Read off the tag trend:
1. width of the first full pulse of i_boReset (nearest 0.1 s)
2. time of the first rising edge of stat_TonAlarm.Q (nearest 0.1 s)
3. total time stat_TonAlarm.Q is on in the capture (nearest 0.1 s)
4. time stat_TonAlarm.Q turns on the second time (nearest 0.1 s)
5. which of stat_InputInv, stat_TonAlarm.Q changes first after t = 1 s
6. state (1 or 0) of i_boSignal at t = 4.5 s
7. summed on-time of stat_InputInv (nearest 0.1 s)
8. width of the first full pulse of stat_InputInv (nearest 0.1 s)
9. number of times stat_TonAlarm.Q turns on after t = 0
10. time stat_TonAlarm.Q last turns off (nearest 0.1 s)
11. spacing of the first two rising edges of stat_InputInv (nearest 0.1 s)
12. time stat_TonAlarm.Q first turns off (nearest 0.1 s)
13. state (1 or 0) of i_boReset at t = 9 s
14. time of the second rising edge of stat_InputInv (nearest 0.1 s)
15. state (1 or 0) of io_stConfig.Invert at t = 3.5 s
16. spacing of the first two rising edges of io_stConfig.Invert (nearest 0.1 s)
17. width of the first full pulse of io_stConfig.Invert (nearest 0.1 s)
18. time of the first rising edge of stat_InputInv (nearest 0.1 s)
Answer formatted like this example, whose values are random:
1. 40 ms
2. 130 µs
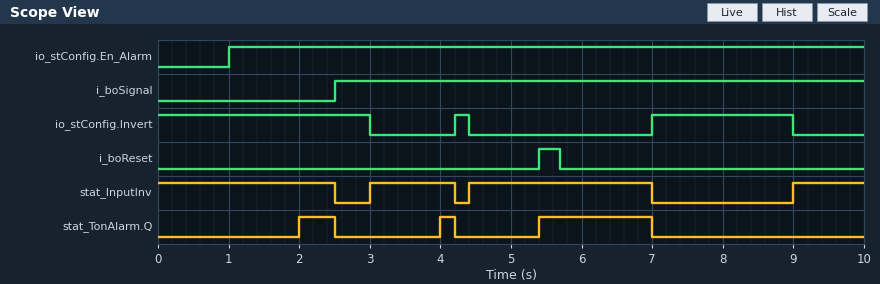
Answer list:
1. 0.3 s
2. 2.0 s
3. 2.3 s
4. 4.0 s
5. stat_TonAlarm.Q
6. 1
7. 7.3 s
8. 1.2 s
9. 3
10. 7.0 s
11. 1.4 s
12. 2.5 s
13. 0
14. 4.4 s
15. 0
16. 2.8 s
17. 0.2 s
18. 3.0 s
